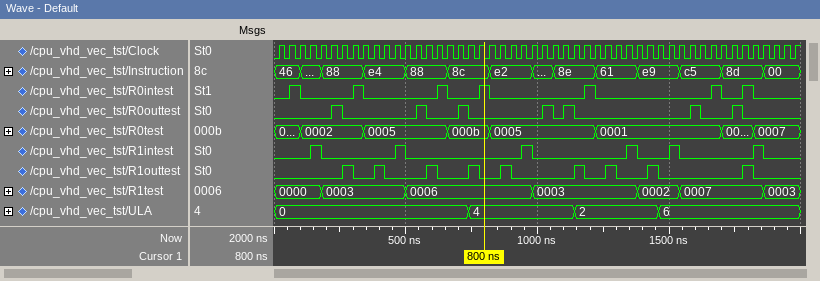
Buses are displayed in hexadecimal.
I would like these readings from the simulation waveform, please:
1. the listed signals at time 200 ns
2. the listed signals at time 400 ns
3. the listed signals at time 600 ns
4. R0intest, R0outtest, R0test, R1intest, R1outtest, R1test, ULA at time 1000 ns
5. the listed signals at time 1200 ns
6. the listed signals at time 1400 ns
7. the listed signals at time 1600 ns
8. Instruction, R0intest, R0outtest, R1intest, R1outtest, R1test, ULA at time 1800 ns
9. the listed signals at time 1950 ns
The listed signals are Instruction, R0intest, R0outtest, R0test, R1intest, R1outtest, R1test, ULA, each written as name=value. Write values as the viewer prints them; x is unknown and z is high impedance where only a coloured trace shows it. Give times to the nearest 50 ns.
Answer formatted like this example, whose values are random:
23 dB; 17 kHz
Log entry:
Instruction=88, R0intest=0, R0outtest=0, R0test=0002, R1intest=0, R1outtest=0, R1test=0003, ULA=0; Instruction=e4, R0intest=0, R0outtest=0, R0test=0005, R1intest=0, R1outtest=1, R1test=0003, ULA=0; Instruction=88, R0intest=0, R0outtest=0, R0test=0005, R1intest=0, R1outtest=1, R1test=0006, ULA=0; R0intest=0, R0outtest=0, R0test=0005, R1intest=0, R1outtest=0, R1test=0003, ULA=4; Instruction=8e, R0intest=1, R0outtest=0, R0test=0005, R1intest=0, R1outtest=0, R1test=0003, ULA=2; Instruction=e9, R0intest=0, R0outtest=0, R0test=0001, R1intest=0, R1outtest=0, R1test=0002, ULA=2; Instruction=c5, R0intest=0, R0outtest=1, R0test=0001, R1intest=0, R1outtest=0, R1test=0007, ULA=6; Instruction=8d, R0intest=1, R0outtest=0, R1intest=0, R1outtest=1, R1test=0007, ULA=6; Instruction=00, R0intest=0, R0outtest=0, R0test=0007, R1intest=0, R1outtest=0, R1test=0003, ULA=6
